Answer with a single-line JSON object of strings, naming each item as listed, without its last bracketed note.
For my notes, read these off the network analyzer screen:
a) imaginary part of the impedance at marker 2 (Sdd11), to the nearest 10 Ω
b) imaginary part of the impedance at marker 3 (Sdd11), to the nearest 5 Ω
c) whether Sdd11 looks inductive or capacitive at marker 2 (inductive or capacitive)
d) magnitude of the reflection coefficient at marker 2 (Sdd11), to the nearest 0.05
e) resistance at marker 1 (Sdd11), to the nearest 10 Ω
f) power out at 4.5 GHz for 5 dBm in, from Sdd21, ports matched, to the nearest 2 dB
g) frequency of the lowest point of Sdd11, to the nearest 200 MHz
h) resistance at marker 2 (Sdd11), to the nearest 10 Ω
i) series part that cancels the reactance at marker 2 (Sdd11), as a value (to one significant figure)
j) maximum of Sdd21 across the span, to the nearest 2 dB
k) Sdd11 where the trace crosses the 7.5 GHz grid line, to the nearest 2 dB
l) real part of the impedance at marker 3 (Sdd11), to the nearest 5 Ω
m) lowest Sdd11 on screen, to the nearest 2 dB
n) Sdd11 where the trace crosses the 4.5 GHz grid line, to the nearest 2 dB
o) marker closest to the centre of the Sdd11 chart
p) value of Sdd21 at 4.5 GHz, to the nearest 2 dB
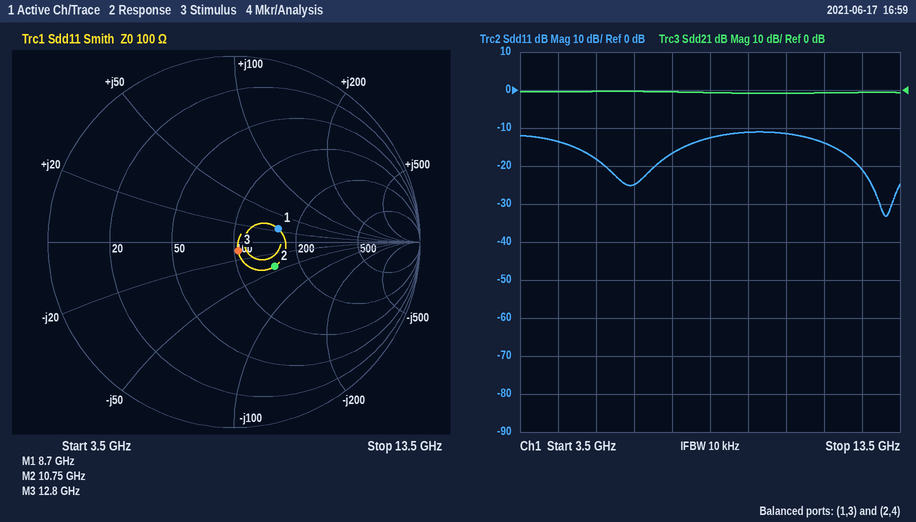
{"imaginary part of the impedance at marker 2 (Sdd11), to the nearest 10 Ω": "-40 Ω", "imaginary part of the impedance at marker 3 (Sdd11), to the nearest 5 Ω": "-10 Ω", "whether Sdd11 looks inductive or capacitive at marker 2": "capacitive", "magnitude of the reflection coefficient at marker 2 (Sdd11), to the nearest 0.05": "0.25", "resistance at marker 1 (Sdd11), to the nearest 10 Ω": "160 Ω", "power out at 4.5 GHz for 5 dBm in, from Sdd21, ports matched, to the nearest 2 dB": "4 dBm", "frequency of the lowest point of Sdd11, to the nearest 200 MHz": "13.2 GHz", "resistance at marker 2 (Sdd11), to the nearest 10 Ω": "150 Ω", "series part that cancels the reactance at marker 2 (Sdd11), as a value": "600 pH", "maximum of Sdd21 across the span, to the nearest 2 dB": "0 dB", "Sdd11 where the trace crosses the 7.5 GHz grid line, to the nearest 2 dB": "-16 dB", "real part of the impedance at marker 3 (Sdd11), to the nearest 5 Ω": "105 Ω", "lowest Sdd11 on screen, to the nearest 2 dB": "-34 dB", "Sdd11 where the trace crosses the 4.5 GHz grid line, to the nearest 2 dB": "-14 dB", "marker closest to the centre of the Sdd11 chart": "marker 3", "value of Sdd21 at 4.5 GHz, to the nearest 2 dB": "0 dB"}
